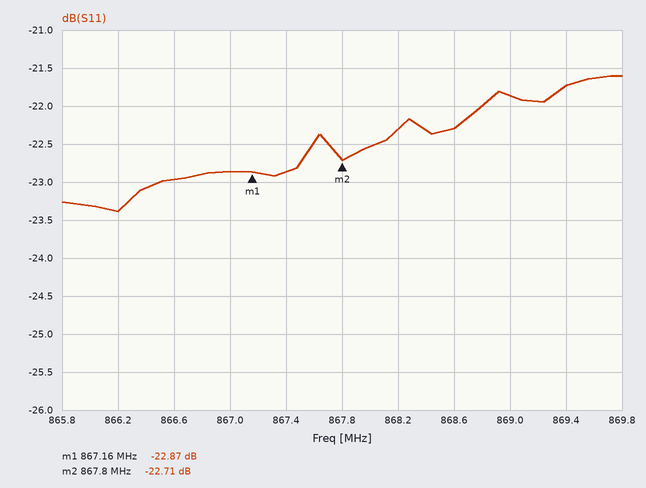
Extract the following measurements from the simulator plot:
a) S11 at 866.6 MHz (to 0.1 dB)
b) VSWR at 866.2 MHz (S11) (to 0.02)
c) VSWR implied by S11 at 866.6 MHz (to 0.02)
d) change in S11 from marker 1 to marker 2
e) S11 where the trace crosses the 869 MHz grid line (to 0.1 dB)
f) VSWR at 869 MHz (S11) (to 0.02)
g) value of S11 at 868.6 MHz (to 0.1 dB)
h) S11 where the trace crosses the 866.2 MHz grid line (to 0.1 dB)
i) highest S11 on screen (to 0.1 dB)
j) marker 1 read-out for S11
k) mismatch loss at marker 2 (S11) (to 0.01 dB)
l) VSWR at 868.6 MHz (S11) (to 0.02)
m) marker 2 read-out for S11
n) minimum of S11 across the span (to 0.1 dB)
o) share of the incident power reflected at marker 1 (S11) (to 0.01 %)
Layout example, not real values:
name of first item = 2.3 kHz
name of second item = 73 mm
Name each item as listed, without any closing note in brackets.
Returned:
S11 at 866.6 MHz = -23.0 dB
VSWR at 866.2 MHz (S11) = 1.14
VSWR implied by S11 at 866.6 MHz = 1.16
change in S11 from marker 1 to marker 2 = 0.16 dB
S11 where the trace crosses the 869 MHz grid line = -21.9 dB
VSWR at 869 MHz (S11) = 1.18
value of S11 at 868.6 MHz = -22.3 dB
S11 where the trace crosses the 866.2 MHz grid line = -23.4 dB
highest S11 on screen = -21.6 dB
marker 1 read-out for S11 = -22.87 dB
mismatch loss at marker 2 (S11) = 0.02 dB
VSWR at 868.6 MHz (S11) = 1.16
marker 2 read-out for S11 = -22.71 dB
minimum of S11 across the span = -23.4 dB
share of the incident power reflected at marker 1 (S11) = 0.52 %
